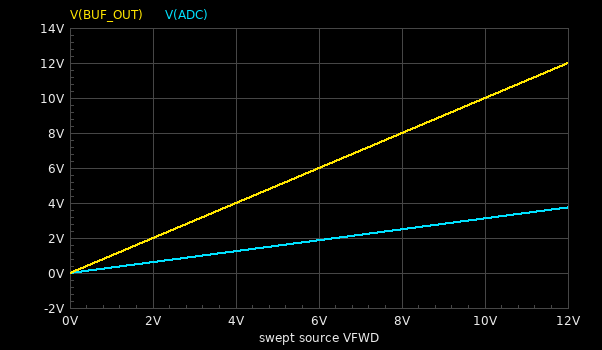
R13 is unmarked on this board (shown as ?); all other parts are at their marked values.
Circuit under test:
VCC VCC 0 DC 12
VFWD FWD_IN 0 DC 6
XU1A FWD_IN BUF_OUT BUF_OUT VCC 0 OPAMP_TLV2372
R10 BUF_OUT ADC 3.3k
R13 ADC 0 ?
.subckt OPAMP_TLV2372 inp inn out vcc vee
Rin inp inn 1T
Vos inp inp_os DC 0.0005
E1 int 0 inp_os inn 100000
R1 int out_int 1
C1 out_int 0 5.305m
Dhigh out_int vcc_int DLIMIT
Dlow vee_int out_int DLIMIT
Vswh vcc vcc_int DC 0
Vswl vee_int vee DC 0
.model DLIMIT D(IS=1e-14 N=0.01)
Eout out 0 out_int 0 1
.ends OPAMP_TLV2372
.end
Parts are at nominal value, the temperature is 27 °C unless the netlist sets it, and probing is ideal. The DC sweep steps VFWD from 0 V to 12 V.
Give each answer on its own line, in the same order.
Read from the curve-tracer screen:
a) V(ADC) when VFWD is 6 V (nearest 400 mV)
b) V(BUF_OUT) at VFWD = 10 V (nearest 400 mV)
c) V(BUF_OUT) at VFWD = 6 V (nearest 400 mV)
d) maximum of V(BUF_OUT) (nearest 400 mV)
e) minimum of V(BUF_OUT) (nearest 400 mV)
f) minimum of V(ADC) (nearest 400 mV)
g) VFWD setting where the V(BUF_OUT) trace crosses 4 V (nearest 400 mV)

2.0 V
10.0 V
6.0 V
12.0 V
0 V
0 V
4.0 V
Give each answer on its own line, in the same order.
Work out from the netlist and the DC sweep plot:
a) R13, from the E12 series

1.5 kΩ
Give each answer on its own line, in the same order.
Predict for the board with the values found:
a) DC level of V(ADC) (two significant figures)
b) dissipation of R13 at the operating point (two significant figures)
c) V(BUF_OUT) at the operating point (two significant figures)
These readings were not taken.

1.9 V
2.3 mW
6.0 V
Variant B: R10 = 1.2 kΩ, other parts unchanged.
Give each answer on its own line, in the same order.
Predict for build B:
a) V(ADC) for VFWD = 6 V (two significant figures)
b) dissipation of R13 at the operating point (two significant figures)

3.3 V
7.4 mW
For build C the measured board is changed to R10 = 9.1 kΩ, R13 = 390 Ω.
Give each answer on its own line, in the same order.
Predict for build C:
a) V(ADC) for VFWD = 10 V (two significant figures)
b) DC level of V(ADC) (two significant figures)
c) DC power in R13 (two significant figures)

410 mV
250 mV
160 µW
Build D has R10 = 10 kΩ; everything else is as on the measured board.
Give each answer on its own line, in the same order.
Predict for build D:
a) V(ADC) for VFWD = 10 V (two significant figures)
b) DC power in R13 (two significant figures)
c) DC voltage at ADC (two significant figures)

1.3 V
410 µW
780 mV
